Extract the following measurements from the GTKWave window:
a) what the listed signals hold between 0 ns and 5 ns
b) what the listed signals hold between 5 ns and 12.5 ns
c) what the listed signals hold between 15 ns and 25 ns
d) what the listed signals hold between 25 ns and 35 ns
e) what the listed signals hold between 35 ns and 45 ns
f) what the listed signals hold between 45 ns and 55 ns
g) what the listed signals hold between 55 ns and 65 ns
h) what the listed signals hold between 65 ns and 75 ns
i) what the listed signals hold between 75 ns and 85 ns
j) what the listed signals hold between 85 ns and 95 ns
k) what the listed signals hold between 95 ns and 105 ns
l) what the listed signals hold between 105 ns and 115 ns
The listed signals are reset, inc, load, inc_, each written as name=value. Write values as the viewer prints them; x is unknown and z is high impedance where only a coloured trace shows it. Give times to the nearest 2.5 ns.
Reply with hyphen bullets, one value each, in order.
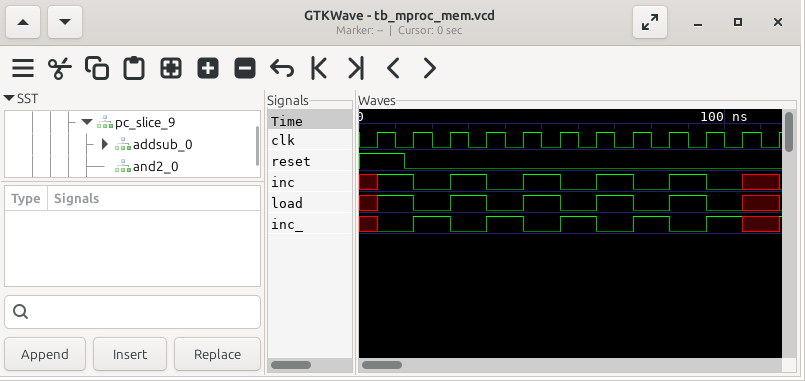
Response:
- reset=1, inc=x, load=x, inc_=x
- reset=1, inc=1, load=1, inc_=0
- reset=0, inc=0, load=0, inc_=1
- reset=0, inc=1, load=1, inc_=0
- reset=0, inc=0, load=0, inc_=1
- reset=0, inc=1, load=1, inc_=0
- reset=0, inc=0, load=0, inc_=1
- reset=0, inc=1, load=1, inc_=0
- reset=0, inc=0, load=0, inc_=1
- reset=0, inc=1, load=1, inc_=0
- reset=0, inc=0, load=0, inc_=1
- reset=0, inc=x, load=x, inc_=x
